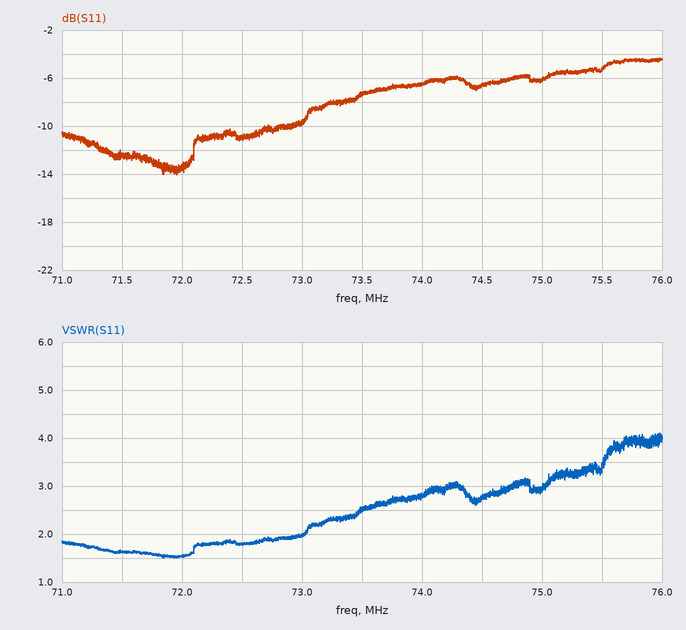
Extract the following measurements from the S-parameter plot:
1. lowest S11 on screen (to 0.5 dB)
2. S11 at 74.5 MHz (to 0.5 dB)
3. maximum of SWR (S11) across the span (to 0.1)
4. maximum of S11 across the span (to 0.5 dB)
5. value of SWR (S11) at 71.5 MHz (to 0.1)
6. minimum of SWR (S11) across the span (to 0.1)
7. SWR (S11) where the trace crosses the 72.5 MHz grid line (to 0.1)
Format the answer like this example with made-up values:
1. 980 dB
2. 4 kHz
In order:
1. -14.0 dB
2. -6.5 dB
3. 4.1
4. -4.5 dB
5. 1.6
6. 1.5
7. 1.8
